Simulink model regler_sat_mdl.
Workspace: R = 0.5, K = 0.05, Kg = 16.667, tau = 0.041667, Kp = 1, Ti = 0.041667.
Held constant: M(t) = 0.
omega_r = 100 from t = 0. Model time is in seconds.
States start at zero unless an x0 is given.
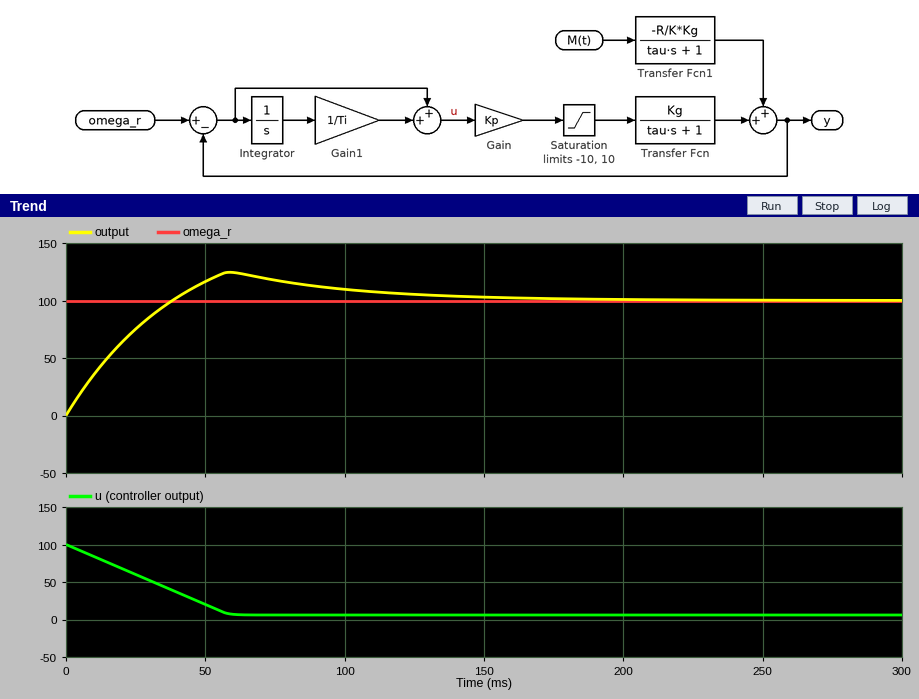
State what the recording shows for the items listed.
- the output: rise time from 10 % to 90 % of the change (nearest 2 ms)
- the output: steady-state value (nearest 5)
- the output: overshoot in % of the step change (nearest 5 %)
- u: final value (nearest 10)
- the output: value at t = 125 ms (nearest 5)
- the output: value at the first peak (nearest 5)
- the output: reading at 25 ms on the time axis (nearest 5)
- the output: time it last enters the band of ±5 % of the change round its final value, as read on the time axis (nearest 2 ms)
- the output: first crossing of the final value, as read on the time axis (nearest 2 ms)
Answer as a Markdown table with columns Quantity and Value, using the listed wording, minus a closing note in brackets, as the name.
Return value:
| Quantity | Value |
|---|---|
| the output: rise time from 10 % to 90 % of the change | 30 ms |
| the output: steady-state value | 100 |
| the output: overshoot in % of the step change | 25 % |
| u: final value | 10 |
| the output: value at t = 125 ms | 105 |
| the output: value at the first peak | 125 |
| the output: reading at 25 ms on the time axis | 75 |
| the output: time it last enters the band of ±5 % of the change round its final value, as read on the time axis | 128 ms |
| the output: first crossing of the final value, as read on the time axis | 38 ms |
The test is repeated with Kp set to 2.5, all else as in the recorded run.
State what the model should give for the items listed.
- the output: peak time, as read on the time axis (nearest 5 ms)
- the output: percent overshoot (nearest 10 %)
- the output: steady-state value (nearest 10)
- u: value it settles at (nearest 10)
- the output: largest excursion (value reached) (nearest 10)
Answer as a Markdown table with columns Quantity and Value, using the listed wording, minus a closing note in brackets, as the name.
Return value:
| Quantity | Value |
|---|---|
| the output: peak time, as read on the time axis | 60 ms |
| the output: percent overshoot | 30 % |
| the output: steady-state value | 100 |
| u: value it settles at | 0 |
| the output: largest excursion (value reached) | 130 |
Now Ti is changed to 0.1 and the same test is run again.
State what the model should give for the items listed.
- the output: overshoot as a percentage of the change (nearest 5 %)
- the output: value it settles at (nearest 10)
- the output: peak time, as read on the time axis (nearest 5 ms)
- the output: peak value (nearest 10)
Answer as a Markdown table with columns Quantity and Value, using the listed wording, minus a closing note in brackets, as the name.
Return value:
| Quantity | Value |
|---|---|
| the output: overshoot as a percentage of the change | 10 % |
| the output: value it settles at | 100 |
| the output: peak time, as read on the time axis | 50 ms |
| the output: peak value | 110 |
